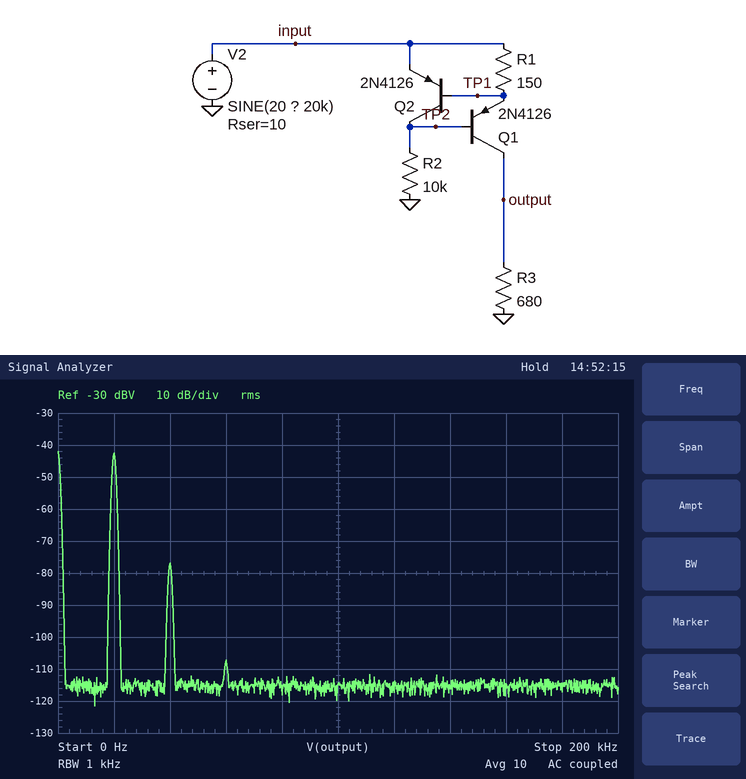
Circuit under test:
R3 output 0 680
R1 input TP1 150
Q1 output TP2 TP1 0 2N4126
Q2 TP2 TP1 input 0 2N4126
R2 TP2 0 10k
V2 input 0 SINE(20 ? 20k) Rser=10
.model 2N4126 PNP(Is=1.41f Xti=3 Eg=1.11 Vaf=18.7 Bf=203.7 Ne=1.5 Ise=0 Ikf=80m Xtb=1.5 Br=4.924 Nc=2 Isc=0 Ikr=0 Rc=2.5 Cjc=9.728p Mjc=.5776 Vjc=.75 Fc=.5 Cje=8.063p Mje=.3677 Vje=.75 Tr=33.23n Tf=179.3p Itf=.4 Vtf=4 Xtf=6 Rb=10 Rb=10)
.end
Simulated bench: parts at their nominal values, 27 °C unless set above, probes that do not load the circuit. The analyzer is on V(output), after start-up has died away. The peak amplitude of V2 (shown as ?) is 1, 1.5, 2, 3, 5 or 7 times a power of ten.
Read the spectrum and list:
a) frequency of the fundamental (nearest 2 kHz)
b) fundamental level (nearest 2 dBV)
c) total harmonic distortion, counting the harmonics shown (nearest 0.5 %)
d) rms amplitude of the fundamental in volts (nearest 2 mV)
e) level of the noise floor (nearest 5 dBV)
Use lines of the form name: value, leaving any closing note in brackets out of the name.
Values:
frequency of the fundamental: 20 kHz
fundamental level: -42 dBV
total harmonic distortion, counting the harmonics shown: 2.0 %
rms amplitude of the fundamental in volts: 8 mV
level of the noise floor: -115 dBV
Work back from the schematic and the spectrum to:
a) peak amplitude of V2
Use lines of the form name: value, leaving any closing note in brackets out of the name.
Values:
peak amplitude of V2: 1.5 V
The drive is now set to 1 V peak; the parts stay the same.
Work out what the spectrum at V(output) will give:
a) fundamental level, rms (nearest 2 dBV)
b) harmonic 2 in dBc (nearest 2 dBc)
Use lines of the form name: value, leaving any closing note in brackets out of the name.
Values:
fundamental level, rms: -46 dBV
harmonic 2 in dBc: -38 dBc
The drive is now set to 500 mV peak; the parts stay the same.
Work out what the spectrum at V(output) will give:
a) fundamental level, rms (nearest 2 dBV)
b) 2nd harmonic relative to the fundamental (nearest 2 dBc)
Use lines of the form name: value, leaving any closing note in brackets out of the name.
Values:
fundamental level, rms: -52 dBV
2nd harmonic relative to the fundamental: -44 dBc
